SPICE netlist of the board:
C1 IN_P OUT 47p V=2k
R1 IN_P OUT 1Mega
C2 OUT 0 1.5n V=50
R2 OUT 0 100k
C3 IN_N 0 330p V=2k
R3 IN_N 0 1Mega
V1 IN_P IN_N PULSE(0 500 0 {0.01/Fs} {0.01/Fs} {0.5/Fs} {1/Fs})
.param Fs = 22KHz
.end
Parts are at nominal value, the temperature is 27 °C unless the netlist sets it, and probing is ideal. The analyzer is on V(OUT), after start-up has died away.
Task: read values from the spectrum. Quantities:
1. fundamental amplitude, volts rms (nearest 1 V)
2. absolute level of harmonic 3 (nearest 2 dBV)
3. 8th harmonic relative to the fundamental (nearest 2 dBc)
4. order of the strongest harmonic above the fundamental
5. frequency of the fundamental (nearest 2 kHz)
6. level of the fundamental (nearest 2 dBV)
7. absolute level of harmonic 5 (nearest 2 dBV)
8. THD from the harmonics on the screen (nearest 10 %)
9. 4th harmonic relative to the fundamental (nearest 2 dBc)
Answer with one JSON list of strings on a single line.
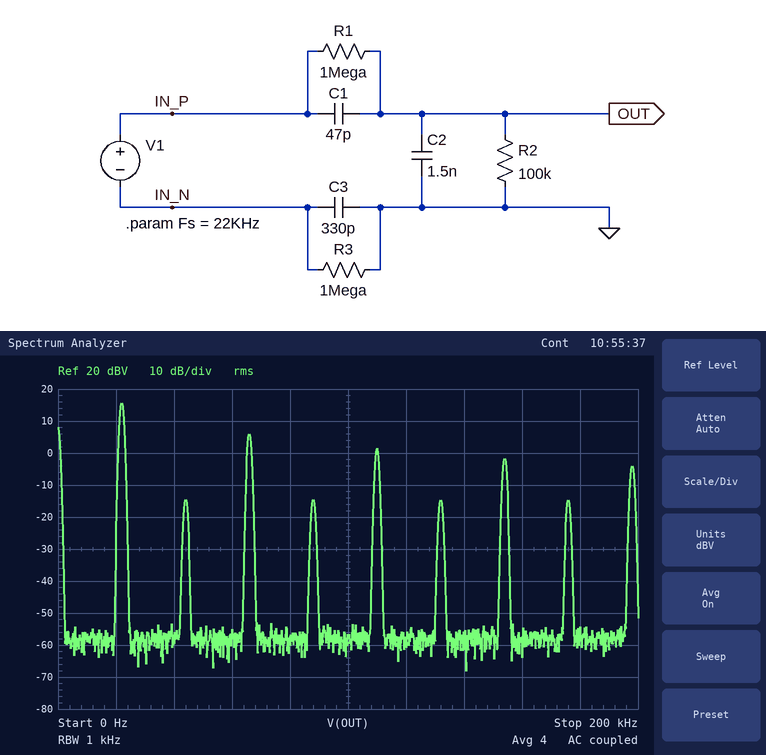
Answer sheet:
["6 V", "6 dBV", "-30 dBc", "3", "22 kHz", "16 dBV", "2 dBV", "40 %", "-30 dBc"]
